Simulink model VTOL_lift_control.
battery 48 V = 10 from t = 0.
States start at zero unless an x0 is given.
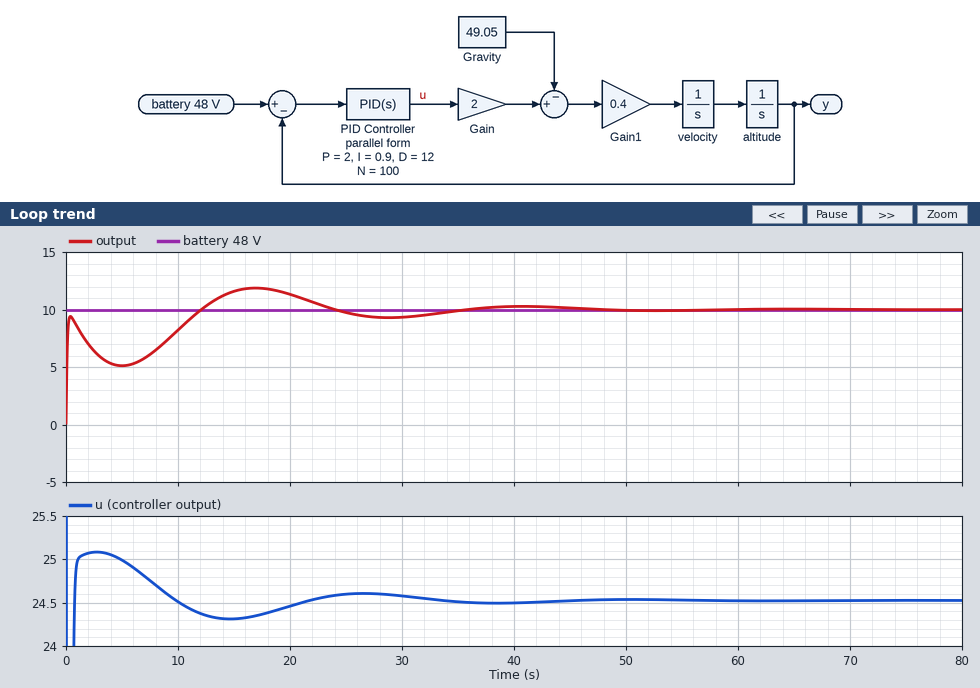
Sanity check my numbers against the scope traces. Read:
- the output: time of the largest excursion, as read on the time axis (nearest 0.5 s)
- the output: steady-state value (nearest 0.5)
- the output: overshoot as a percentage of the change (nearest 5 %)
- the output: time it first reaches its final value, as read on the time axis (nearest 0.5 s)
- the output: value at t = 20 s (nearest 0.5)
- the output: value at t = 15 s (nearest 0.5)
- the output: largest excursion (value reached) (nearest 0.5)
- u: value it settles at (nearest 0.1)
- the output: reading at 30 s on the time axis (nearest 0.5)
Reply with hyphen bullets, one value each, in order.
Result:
- 17.0 s
- 10.0
- 20 %
- 12.0 s
- 11.5
- 11.5
- 12.0
- 24.5
- 9.5
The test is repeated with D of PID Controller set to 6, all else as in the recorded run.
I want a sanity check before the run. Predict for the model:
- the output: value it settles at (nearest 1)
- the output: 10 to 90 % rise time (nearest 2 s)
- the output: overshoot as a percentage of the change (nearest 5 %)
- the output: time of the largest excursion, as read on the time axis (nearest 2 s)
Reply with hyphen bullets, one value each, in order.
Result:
- 10
- 8 s
- 15 %
- 12 s
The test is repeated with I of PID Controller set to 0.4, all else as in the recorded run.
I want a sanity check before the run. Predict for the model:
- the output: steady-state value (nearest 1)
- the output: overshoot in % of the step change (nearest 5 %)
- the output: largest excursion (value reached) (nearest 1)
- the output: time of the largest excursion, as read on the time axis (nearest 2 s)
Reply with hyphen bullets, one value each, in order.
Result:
- 10
- 15 %
- 11
- 26 s
